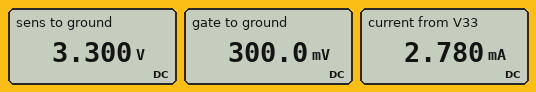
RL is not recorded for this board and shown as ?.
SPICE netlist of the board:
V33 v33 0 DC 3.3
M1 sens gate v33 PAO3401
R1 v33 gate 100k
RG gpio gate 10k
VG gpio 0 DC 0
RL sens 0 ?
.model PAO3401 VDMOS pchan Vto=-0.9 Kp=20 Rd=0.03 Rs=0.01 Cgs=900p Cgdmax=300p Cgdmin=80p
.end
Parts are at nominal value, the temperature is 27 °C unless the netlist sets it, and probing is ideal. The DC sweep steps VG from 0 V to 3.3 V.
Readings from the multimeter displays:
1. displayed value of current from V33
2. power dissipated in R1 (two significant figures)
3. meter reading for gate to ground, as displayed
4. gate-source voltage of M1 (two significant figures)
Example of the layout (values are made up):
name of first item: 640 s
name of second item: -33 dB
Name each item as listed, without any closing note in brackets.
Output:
displayed value of current from V33: 2.780 mA
power dissipated in R1: 90 µW
meter reading for gate to ground, as displayed: 300.0 mV
gate-source voltage of M1: -3.0 V
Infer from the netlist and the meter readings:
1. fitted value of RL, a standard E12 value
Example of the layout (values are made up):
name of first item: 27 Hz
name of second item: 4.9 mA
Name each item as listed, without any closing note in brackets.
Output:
fitted value of RL, a standard E12 value: 1.2 kΩ
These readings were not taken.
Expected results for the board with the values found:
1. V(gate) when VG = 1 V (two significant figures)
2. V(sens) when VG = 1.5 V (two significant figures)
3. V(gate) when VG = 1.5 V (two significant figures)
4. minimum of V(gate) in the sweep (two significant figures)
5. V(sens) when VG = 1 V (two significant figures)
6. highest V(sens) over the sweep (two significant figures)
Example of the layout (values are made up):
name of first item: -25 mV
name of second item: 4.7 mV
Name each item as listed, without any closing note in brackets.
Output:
V(gate) when VG = 1 V: 1.2 V
V(sens) when VG = 1.5 V: 3.3 V
V(gate) when VG = 1.5 V: 1.7 V
minimum of V(gate) in the sweep: 300 mV
V(sens) when VG = 1 V: 3.3 V
highest V(sens) over the sweep: 3.3 V
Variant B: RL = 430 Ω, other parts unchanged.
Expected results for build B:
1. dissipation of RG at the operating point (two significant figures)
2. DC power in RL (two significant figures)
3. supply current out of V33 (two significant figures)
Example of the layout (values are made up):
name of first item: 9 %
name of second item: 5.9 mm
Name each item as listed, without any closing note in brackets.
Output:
dissipation of RG at the operating point: 9.0 µW
DC power in RL: 25 mW
supply current out of V33: 7.7 mA
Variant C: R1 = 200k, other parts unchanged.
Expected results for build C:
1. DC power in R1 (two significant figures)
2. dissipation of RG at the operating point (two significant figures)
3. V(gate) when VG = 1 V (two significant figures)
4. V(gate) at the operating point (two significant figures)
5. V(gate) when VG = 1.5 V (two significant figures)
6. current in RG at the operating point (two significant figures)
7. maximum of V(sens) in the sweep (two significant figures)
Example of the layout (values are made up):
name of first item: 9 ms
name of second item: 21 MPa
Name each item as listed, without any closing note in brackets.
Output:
DC power in R1: 49 µW
dissipation of RG at the operating point: 2.5 µW
V(gate) when VG = 1 V: 1.1 V
V(gate) at the operating point: 160 mV
V(gate) when VG = 1.5 V: 1.6 V
current in RG at the operating point: 16 µA
maximum of V(sens) in the sweep: 3.3 V
